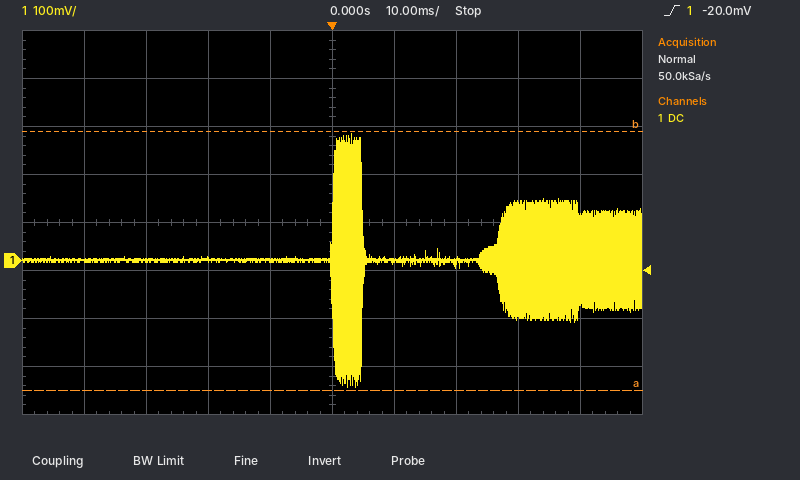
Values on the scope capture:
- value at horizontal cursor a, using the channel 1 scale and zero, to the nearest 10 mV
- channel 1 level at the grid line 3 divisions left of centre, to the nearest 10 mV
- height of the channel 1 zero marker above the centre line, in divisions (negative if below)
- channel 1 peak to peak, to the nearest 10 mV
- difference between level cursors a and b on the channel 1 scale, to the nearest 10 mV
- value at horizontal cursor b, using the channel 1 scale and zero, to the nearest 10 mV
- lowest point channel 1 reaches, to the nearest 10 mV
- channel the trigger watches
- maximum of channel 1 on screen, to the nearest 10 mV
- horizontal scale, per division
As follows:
-270 mV
0 mV
-0.8 div
530 mV
540 mV
270 mV
-260 mV
channel 1
270 mV
10 ms
